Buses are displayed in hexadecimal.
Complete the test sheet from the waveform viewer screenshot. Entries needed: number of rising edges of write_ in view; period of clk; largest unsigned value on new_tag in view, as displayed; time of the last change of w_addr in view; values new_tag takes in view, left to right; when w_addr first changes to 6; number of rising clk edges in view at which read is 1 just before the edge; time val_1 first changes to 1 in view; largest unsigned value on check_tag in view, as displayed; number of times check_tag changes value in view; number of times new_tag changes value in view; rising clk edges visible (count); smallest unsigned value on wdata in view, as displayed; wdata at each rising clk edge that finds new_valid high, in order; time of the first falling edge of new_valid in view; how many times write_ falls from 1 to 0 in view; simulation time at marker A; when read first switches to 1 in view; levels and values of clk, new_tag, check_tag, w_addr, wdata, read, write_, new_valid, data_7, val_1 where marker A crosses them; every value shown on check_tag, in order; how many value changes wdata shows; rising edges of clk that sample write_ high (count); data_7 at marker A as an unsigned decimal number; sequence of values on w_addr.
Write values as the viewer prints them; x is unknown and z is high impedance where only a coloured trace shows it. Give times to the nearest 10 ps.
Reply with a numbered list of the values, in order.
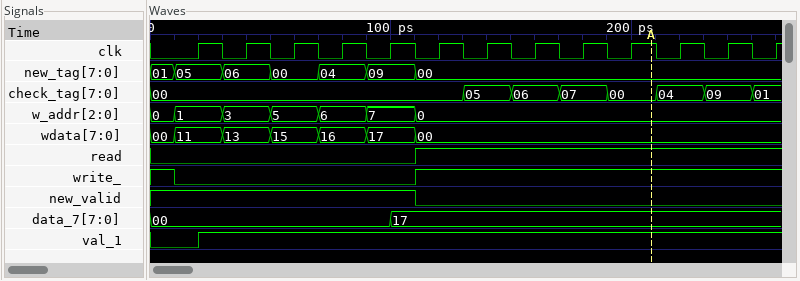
1. 1
2. 20 ps
3. 09
4. 110 ps
5. 01, 05, 06, 00, 04, 09, 00
6. 70 ps
7. 8
8. 20 ps
9. 09
10. 7
11. 6
12. 13
13. 00
14. 11, 13, 15, 16, 17
15. 110 ps
16. 1
17. 210 ps
18. 110 ps
19. clk=1, new_tag=00, check_tag=00, w_addr=0, wdata=00, read=1, write_=1, new_valid=0, data_7=17, val_1=1
20. 00, 05, 06, 07, 00, 04, 09, 01
21. 6
22. 8
23. 23
24. 0, 1, 3, 5, 6, 7, 0
